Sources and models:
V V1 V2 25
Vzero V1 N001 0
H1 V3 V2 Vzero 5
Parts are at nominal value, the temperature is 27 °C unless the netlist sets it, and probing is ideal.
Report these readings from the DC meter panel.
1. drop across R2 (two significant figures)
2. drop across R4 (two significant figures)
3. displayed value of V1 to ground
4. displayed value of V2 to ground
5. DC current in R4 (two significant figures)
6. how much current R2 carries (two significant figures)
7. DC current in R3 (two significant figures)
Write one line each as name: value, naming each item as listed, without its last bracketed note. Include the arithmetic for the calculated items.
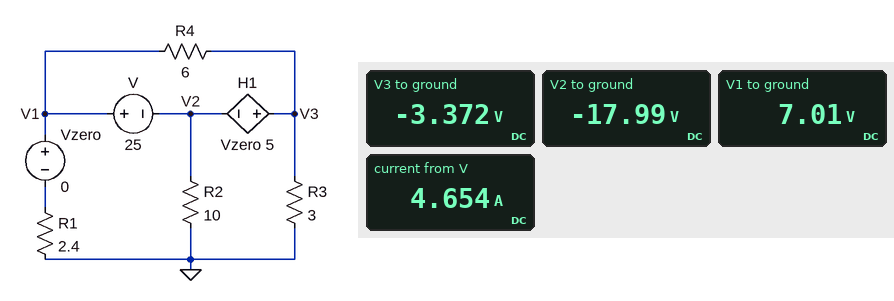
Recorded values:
drop across R2: 0 V - (-17.99 V) = 18 V
drop across R4: 7.01 V - (-3.372 V) = 10 V
displayed value of V1 to ground: 7.01 V
displayed value of V2 to ground: -17.99 V
DC current in R4: (7.01 V - (-3.372 V)) / 6 Ω = 1.7 A
how much current R2 carries: (0 V - (-17.99 V)) / 10 Ω = 1.8 A
DC current in R3: (0 V - (-3.372 V)) / 3 Ω = 1.1 A
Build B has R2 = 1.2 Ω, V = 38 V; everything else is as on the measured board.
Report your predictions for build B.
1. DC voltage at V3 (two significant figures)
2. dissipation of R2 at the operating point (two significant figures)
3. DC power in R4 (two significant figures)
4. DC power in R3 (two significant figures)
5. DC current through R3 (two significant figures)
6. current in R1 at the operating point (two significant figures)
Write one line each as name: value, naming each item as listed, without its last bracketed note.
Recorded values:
DC voltage at V3: 22 V
dissipation of R2 at the operating point: 290 W
DC power in R4: 1.1 W
DC power in R3: 160 W
DC current through R3: 7.3 A
current in R1 at the operating point: 8.1 A
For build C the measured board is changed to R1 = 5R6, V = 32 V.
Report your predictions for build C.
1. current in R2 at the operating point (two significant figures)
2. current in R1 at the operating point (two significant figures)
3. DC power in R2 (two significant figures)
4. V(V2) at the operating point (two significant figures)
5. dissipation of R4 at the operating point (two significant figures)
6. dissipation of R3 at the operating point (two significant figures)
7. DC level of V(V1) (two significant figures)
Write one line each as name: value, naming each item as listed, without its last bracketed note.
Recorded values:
current in R2 at the operating point: 1.7 A
current in R1 at the operating point: 2.7 A
DC power in R2: 28 W
V(V2) at the operating point: -17 V
dissipation of R4 at the operating point: 56 W
dissipation of R3 at the operating point: 3.3 W
DC level of V(V1): 15 V
